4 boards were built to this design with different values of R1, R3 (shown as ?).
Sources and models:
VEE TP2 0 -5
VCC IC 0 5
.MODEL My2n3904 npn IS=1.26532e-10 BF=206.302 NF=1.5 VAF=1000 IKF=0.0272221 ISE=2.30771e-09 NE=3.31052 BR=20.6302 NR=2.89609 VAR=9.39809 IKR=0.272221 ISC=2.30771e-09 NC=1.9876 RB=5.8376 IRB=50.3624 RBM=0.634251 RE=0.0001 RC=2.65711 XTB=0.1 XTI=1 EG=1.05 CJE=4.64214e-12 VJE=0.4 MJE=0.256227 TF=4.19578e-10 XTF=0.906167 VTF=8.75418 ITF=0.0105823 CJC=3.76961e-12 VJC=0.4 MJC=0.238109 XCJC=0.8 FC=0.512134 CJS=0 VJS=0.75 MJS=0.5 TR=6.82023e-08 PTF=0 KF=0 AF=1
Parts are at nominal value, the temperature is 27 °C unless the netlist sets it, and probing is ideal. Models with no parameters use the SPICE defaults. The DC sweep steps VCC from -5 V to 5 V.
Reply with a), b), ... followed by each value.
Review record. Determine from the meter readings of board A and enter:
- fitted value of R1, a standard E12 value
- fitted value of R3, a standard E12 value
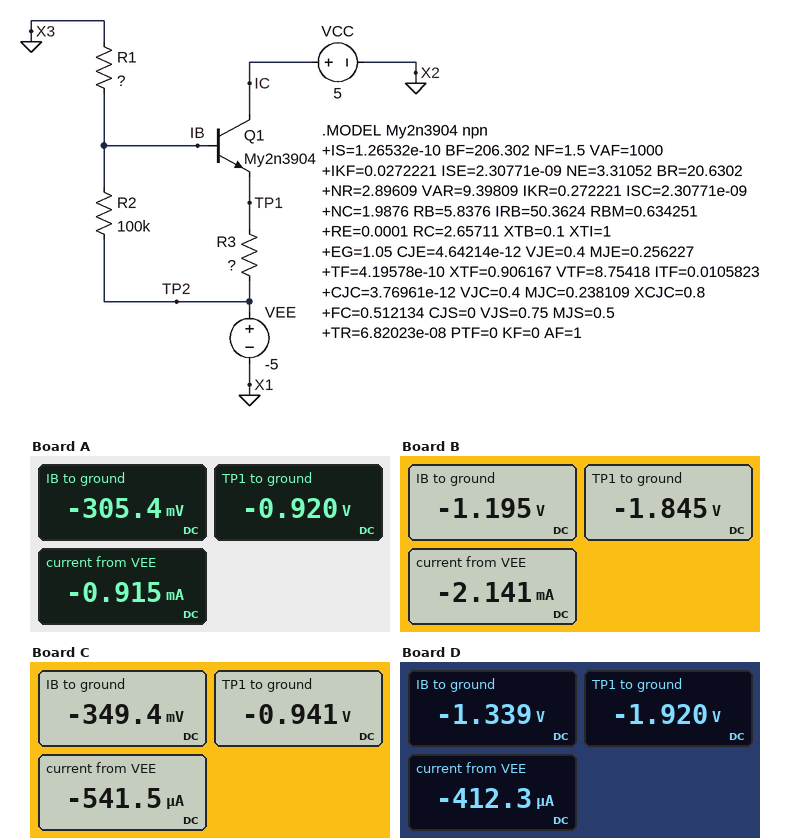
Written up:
a) 5.6 kΩ
b) 4.7 kΩ
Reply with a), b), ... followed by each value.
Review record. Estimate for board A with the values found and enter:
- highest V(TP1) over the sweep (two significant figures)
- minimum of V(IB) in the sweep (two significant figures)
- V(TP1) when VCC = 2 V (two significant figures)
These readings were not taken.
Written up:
a) -920 mV
b) -4.3 V
c) -920 mV
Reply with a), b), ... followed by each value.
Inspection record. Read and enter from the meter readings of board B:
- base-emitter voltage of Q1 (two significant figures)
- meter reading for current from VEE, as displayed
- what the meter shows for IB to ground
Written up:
a) 650 mV
b) -2.141 mA
c) -1.195 V
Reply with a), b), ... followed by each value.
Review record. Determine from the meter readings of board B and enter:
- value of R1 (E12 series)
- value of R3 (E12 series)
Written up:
a) 22 kΩ
b) 1.5 kΩ
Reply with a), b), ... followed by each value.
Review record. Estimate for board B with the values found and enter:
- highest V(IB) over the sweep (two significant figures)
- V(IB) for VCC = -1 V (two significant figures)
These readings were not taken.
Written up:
a) -1.2 V
b) -1.2 V
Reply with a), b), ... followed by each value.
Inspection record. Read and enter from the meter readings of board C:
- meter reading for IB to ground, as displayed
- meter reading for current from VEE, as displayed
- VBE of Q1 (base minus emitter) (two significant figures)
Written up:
a) -349.4 mV
b) -541.5 µA
c) 590 mV
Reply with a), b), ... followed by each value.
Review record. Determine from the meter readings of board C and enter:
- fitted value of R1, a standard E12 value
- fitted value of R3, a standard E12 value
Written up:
a) 6.8 kΩ
b) 8.2 kΩ
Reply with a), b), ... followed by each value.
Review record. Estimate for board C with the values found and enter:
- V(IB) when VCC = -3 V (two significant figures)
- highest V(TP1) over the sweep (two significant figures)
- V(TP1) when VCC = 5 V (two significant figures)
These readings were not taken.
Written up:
a) -2.4 V
b) -940 mV
c) -940 mV
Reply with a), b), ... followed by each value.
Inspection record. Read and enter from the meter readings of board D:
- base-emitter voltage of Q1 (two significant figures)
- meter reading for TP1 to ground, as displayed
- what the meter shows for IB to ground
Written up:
a) 580 mV
b) -1.920 V
c) -1.339 V
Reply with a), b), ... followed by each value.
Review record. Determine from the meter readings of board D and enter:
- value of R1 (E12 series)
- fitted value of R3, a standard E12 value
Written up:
a) 33 kΩ
b) 8.2 kΩ
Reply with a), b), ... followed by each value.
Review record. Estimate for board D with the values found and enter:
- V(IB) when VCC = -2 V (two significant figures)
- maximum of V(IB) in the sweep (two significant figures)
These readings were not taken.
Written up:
a) -1.6 V
b) -1.3 V
